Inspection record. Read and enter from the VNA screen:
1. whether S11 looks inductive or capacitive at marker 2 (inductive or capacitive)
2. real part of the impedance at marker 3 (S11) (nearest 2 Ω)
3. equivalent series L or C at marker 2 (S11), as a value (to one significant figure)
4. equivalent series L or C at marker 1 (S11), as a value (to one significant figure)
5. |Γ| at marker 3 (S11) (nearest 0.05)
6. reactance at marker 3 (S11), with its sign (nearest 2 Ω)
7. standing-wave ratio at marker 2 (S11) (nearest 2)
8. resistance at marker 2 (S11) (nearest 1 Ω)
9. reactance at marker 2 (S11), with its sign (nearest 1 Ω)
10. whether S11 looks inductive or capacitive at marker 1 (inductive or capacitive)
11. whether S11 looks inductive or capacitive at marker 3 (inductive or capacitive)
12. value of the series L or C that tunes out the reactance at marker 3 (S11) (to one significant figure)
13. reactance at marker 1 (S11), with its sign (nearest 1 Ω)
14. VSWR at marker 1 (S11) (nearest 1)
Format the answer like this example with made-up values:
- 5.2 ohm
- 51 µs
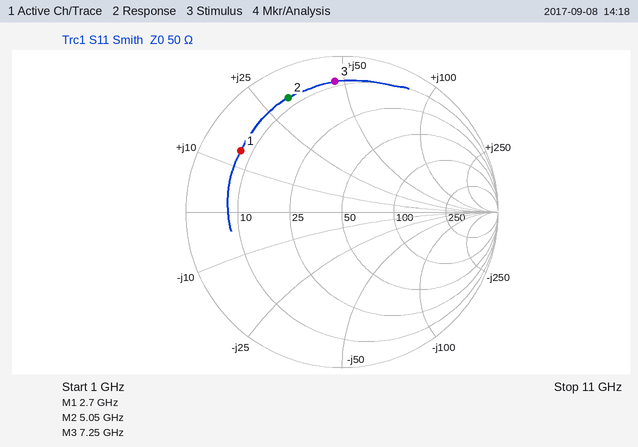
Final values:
- inductive
- 8 Ω
- 1.0 nH
- 800 pH
- 0.85
- +46 Ω
- 10
- 7 Ω
- +31 Ω
- inductive
- inductive
- 500 fF
- +14 Ω
- 7
